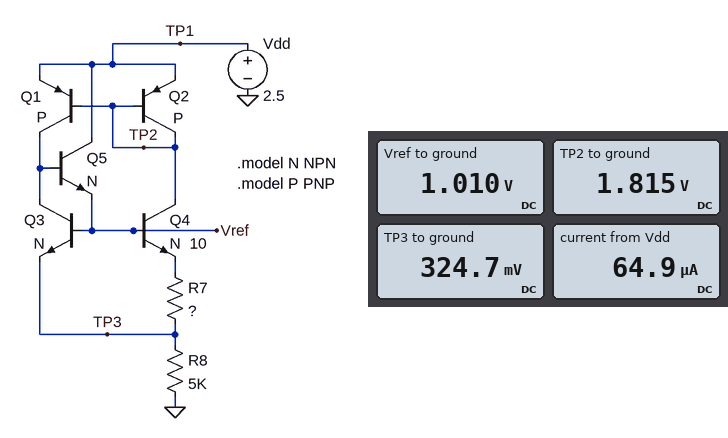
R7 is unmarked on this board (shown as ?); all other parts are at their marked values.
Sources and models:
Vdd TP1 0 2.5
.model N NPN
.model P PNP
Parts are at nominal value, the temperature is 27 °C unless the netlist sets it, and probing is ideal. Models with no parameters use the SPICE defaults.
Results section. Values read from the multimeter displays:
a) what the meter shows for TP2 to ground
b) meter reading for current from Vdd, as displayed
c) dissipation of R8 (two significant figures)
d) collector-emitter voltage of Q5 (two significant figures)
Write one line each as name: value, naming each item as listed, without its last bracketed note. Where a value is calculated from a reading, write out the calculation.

what the meter shows for TP2 to ground: 1.815 V
meter reading for current from Vdd, as displayed: 64.9 µA
dissipation of R8: (324.7 mV)^2 / 5 kΩ = 21 µW
collector-emitter voltage of Q5: 2.5 V - 1.01 V = 1.5 V
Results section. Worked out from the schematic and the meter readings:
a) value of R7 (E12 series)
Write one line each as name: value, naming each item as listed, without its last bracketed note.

value of R7: 1.8 kΩ
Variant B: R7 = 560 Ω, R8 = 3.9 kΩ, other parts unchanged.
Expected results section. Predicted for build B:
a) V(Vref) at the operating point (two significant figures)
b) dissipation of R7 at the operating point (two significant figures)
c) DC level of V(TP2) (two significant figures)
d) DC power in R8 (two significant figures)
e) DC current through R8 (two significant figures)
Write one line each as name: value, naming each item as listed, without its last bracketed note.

V(Vref) at the operating point: 1.5 V
dissipation of R7 at the operating point: 6.2 µW
DC level of V(TP2): 1.8 V
DC power in R8: 170 µW
DC current through R8: 210 µA
